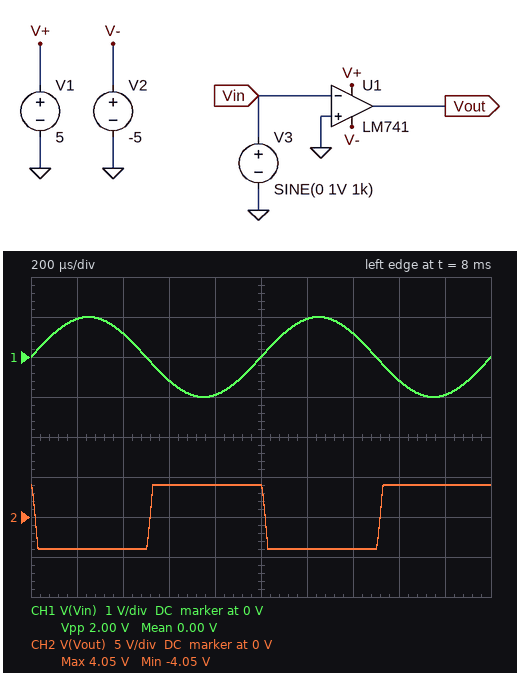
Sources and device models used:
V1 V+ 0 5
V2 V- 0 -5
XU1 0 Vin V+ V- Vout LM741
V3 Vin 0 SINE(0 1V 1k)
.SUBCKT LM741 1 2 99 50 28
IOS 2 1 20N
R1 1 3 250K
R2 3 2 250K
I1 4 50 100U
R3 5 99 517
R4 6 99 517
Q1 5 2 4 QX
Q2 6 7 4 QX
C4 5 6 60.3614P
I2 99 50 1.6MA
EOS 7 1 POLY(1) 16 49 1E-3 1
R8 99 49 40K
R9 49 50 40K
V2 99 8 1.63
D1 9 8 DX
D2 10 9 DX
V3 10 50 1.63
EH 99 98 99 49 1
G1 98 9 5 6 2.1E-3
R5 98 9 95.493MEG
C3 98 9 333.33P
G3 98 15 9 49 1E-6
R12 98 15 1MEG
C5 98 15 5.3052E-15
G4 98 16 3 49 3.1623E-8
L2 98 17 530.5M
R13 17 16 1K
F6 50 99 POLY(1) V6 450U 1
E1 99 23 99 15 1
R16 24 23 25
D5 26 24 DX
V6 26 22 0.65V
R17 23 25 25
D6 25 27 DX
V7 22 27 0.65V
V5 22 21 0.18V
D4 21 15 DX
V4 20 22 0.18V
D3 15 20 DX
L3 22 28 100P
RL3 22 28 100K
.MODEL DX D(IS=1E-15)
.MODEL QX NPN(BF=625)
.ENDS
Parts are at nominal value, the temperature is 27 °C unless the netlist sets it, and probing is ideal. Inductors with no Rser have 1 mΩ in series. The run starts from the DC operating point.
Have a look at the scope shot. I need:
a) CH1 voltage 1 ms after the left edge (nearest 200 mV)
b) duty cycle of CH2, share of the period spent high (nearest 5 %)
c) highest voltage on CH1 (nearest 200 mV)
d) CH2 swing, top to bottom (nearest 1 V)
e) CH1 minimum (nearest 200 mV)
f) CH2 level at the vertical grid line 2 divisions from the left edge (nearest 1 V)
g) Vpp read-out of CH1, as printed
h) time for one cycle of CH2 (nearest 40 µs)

0 V
50 %
1.0 V
8 V
-1.0 V
-4 V
2.00 V
1.00 ms
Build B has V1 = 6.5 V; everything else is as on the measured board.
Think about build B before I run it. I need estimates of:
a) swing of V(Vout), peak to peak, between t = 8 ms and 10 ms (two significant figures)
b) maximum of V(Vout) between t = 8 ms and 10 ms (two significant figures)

9.6 V
5.5 V
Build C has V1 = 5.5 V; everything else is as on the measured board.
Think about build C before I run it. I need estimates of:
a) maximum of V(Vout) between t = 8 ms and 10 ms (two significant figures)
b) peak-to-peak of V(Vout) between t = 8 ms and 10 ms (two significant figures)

4.5 V
8.6 V
